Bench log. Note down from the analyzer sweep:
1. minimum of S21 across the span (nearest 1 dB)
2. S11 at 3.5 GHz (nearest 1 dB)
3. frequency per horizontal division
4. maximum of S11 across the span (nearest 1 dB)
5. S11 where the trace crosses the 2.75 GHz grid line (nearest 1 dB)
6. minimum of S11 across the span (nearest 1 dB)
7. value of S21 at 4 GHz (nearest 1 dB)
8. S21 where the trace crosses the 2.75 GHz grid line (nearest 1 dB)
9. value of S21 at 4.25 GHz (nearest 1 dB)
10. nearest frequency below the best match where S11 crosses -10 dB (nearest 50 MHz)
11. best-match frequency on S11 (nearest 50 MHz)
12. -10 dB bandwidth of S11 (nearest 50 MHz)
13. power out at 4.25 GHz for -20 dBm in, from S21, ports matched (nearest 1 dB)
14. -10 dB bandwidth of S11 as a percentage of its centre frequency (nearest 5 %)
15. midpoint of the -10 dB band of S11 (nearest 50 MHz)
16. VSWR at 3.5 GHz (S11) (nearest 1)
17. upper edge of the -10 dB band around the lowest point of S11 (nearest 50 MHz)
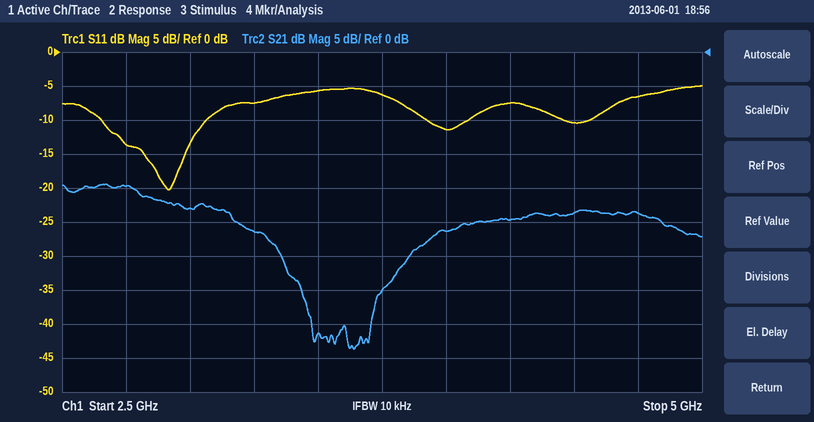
-44 dB
-6 dB
250 MHz
-5 dB
-14 dB
-20 dB
-26 dB
-20 dB
-25 dB
2.65 GHz
2.90 GHz
400 MHz
-45 dBm
15 %
2.85 GHz
3
3.05 GHz
